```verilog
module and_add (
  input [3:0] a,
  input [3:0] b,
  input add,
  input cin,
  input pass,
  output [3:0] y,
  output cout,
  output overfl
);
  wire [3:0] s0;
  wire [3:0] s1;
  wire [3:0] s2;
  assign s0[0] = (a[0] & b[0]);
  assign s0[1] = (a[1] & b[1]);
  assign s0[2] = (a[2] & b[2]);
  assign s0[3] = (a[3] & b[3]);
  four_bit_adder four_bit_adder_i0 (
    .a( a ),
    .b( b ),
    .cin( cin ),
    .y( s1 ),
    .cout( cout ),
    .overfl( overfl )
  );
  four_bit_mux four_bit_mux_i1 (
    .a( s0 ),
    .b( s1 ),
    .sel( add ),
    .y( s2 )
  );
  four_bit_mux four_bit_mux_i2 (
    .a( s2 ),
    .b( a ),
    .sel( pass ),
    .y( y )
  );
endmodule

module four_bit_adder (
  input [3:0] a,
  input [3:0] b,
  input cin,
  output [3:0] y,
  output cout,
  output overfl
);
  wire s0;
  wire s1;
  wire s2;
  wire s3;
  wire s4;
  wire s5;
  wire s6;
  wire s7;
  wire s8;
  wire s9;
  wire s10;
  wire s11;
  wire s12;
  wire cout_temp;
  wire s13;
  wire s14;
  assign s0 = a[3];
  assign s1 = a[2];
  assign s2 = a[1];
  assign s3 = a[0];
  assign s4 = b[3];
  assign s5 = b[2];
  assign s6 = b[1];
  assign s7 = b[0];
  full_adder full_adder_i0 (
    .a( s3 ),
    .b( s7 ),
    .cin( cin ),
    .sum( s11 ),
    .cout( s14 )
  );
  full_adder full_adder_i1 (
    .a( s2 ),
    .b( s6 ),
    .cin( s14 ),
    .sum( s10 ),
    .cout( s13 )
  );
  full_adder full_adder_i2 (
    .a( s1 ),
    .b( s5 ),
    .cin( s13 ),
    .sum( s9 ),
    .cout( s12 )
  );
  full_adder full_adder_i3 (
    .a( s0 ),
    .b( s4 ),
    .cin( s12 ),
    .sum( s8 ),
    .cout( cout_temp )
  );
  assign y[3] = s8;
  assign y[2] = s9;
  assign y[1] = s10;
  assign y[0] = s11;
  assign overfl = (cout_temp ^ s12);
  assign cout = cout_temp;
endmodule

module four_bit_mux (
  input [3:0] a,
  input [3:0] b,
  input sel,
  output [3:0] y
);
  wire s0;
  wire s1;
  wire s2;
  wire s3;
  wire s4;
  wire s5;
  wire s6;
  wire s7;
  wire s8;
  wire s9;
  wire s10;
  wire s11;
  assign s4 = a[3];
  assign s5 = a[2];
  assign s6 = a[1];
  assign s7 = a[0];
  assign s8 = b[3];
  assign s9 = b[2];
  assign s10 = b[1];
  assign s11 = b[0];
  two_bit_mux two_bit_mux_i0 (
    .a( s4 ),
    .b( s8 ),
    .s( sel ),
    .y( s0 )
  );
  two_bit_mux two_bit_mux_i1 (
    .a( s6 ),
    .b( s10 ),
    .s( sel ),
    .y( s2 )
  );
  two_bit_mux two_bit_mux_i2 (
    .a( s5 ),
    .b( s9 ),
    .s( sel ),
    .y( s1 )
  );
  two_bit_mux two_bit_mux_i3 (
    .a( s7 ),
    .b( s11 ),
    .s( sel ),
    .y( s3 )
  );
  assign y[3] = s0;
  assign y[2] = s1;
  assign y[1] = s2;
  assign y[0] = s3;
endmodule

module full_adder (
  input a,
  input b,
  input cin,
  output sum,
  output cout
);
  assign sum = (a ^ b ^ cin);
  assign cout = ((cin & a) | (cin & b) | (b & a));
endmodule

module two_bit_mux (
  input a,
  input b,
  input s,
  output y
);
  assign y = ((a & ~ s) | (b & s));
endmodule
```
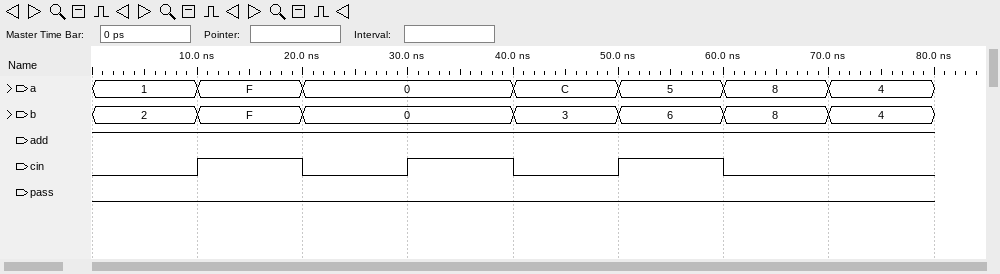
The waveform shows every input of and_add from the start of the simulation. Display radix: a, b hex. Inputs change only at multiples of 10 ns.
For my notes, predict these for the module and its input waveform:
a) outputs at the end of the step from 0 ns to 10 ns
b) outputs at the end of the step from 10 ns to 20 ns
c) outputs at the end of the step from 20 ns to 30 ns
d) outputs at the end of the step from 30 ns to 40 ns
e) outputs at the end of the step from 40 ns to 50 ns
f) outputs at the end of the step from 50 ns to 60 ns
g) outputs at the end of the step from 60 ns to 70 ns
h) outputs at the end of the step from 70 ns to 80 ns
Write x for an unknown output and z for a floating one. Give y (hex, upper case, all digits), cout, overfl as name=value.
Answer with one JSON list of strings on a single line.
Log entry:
["y=3, cout=0, overfl=0", "y=F, cout=1, overfl=0", "y=0, cout=0, overfl=0", "y=1, cout=0, overfl=0", "y=F, cout=0, overfl=0", "y=C, cout=0, overfl=1", "y=0, cout=1, overfl=1", "y=8, cout=0, overfl=1"]
